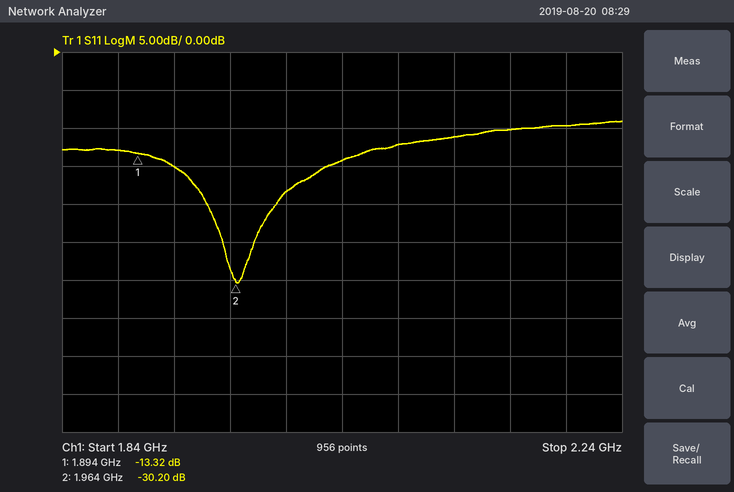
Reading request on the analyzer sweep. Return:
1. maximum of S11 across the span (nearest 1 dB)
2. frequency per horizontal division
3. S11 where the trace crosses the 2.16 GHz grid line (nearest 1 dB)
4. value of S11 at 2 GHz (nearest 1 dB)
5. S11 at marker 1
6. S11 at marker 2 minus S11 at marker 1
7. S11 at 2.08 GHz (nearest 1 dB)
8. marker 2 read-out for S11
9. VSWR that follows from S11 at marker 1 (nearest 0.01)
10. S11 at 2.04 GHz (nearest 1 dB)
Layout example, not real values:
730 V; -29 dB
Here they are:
-9 dB; 40 MHz; -10 dB; -18 dB; -13.32 dB; -16.88 dB; -12 dB; -30.20 dB; 1.55; -14 dB
